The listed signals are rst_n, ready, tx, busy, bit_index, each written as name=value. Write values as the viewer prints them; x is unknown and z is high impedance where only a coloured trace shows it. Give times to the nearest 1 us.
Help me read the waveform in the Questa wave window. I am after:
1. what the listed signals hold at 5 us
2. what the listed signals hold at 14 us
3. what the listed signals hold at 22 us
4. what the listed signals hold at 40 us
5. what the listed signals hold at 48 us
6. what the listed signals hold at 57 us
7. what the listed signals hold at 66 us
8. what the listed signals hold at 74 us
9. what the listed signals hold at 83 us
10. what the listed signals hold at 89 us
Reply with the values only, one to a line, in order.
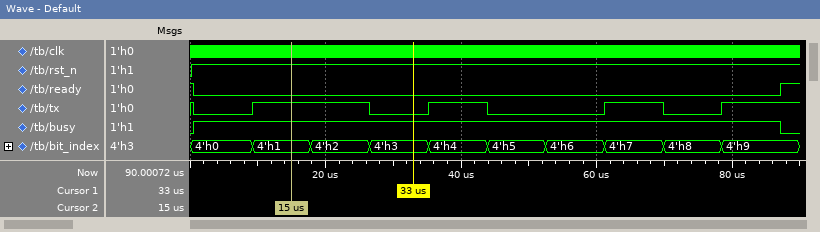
rst_n=1, ready=0, tx=0, busy=1, bit_index=4'h0
rst_n=1, ready=0, tx=1, busy=1, bit_index=4'h1
rst_n=1, ready=0, tx=1, busy=1, bit_index=4'h2
rst_n=1, ready=0, tx=1, busy=1, bit_index=4'h4
rst_n=1, ready=0, tx=0, busy=1, bit_index=4'h5
rst_n=1, ready=0, tx=0, busy=1, bit_index=4'h6
rst_n=1, ready=0, tx=1, busy=1, bit_index=4'h7
rst_n=1, ready=0, tx=0, busy=1, bit_index=4'h8
rst_n=1, ready=0, tx=1, busy=1, bit_index=4'h9
rst_n=1, ready=1, tx=1, busy=0, bit_index=4'h9
